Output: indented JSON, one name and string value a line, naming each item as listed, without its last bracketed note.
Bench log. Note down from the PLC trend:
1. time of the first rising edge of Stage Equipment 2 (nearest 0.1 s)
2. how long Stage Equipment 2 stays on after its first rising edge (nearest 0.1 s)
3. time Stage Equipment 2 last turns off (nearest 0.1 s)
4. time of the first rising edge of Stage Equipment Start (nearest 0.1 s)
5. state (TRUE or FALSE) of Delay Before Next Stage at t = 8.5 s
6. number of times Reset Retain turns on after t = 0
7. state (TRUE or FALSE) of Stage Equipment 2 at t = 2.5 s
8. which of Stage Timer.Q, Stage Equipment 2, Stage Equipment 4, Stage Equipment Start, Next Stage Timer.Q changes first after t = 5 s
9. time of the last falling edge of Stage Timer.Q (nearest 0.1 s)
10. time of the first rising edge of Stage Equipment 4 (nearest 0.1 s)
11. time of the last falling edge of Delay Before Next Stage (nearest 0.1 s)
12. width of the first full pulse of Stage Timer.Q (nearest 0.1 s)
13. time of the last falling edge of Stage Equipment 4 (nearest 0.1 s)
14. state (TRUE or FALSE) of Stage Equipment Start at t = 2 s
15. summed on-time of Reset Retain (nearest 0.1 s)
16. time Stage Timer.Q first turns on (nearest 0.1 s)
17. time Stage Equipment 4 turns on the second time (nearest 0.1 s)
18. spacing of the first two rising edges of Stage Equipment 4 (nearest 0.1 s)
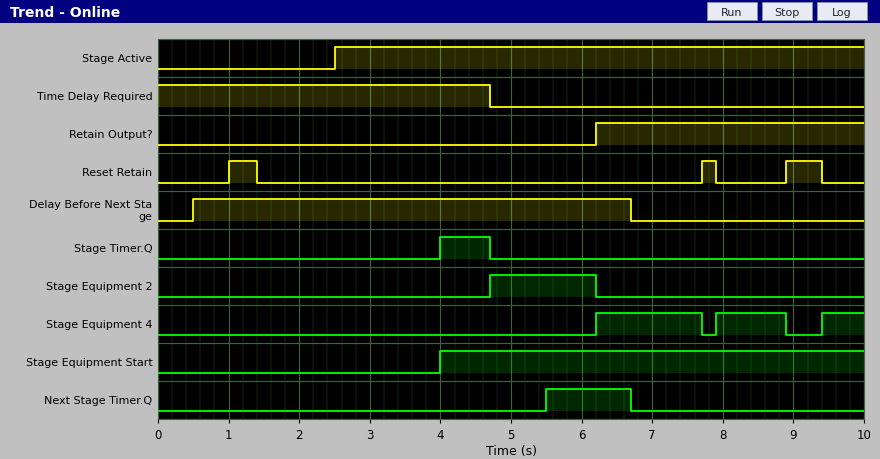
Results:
{
  "time of the first rising edge of Stage Equipment 2": "4.7 s",
  "how long Stage Equipment 2 stays on after its first rising edge": "1.5 s",
  "time Stage Equipment 2 last turns off": "6.2 s",
  "time of the first rising edge of Stage Equipment Start": "4.0 s",
  "state (TRUE or FALSE) of Delay Before Next Stage at t = 8.5 s": "FALSE",
  "number of times Reset Retain turns on after t = 0": "3",
  "state (TRUE or FALSE) of Stage Equipment 2 at t = 2.5 s": "FALSE",
  "which of Stage Timer.Q, Stage Equipment 2, Stage Equipment 4, Stage Equipment Start, Next Stage Timer.Q changes first after t = 5 s": "Next Stage Timer.Q",
  "time of the last falling edge of Stage Timer.Q": "4.7 s",
  "time of the first rising edge of Stage Equipment 4": "6.2 s",
  "time of the last falling edge of Delay Before Next Stage": "6.7 s",
  "width of the first full pulse of Stage Timer.Q": "0.7 s",
  "time of the last falling edge of Stage Equipment 4": "8.9 s",
  "state (TRUE or FALSE) of Stage Equipment Start at t = 2 s": "FALSE",
  "summed on-time of Reset Retain": "1.1 s",
  "time Stage Timer.Q first turns on": "4.0 s",
  "time Stage Equipment 4 turns on the second time": "7.9 s",
  "spacing of the first two rising edges of Stage Equipment 4": "1.7 s"
}
